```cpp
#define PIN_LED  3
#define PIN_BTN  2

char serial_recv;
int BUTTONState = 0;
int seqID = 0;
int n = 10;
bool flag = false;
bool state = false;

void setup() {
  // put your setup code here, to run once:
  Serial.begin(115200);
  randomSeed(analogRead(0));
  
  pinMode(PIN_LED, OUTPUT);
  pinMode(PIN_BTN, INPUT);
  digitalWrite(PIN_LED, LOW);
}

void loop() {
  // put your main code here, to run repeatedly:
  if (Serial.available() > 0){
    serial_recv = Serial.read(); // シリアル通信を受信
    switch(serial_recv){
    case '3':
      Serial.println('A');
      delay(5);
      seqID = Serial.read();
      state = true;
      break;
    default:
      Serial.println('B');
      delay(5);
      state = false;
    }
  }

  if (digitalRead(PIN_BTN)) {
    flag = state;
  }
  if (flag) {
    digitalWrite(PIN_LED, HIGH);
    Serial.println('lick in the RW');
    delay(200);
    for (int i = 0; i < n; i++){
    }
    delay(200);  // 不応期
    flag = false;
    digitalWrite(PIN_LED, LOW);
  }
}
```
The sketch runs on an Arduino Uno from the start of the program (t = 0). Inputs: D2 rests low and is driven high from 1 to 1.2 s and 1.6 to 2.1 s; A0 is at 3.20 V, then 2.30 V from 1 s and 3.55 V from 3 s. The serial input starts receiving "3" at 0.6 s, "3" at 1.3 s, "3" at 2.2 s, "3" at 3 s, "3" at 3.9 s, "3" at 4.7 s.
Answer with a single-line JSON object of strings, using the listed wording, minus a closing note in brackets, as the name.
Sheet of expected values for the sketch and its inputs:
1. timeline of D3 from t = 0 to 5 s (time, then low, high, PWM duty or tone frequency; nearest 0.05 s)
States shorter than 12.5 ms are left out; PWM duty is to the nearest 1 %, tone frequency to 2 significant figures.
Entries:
{"timeline of D3 from t = 0 to 5 s": "0 s low; 1 s high; 1.4 s low; 1.6 s high; 2.4 s low"}
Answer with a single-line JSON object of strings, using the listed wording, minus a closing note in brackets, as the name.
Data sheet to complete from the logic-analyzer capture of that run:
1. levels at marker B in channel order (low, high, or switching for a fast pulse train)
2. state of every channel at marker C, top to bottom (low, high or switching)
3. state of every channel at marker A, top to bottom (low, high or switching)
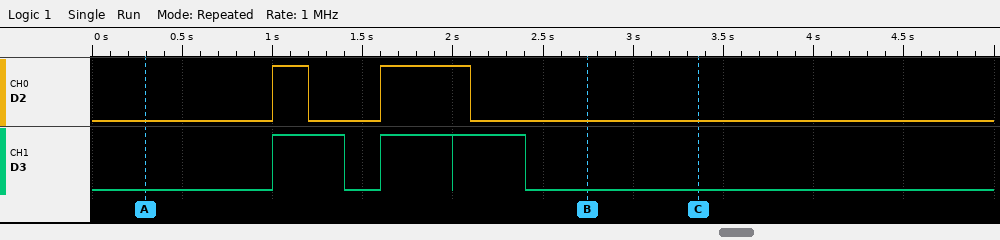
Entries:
{"levels at marker B in channel order": "D2 low, D3 low", "state of every channel at marker C, top to bottom": "D2 low, D3 low", "state of every channel at marker A, top to bottom": "D2 low, D3 low"}
